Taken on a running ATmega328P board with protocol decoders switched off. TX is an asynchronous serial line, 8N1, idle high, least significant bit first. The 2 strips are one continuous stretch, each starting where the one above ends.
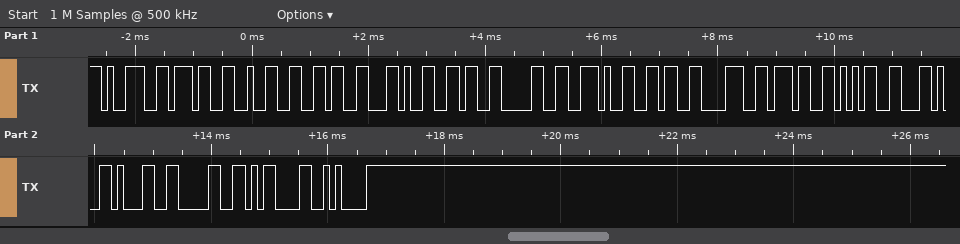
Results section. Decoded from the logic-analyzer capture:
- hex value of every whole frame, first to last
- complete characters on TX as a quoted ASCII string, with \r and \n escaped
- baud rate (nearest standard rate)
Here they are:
39 37 32 36 2C 36 30 2E 36 38 37 35 2C 31 30 0D 0A
"9726,60.6875,10\r\n"
9600 baud
